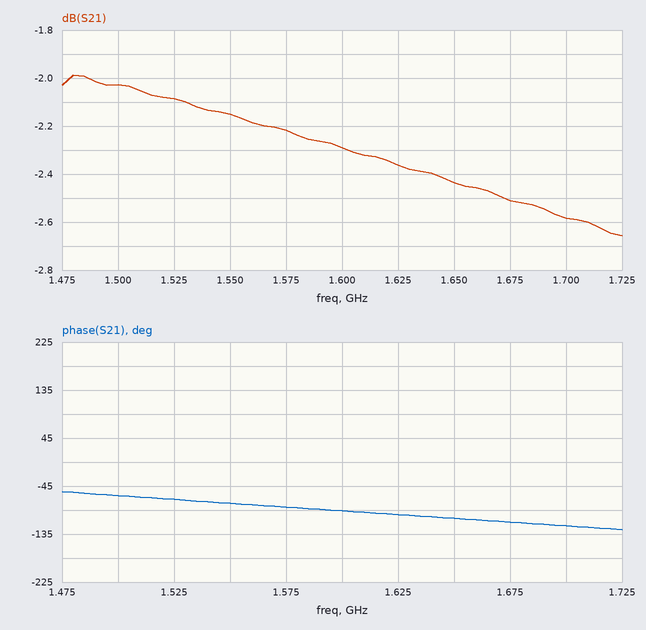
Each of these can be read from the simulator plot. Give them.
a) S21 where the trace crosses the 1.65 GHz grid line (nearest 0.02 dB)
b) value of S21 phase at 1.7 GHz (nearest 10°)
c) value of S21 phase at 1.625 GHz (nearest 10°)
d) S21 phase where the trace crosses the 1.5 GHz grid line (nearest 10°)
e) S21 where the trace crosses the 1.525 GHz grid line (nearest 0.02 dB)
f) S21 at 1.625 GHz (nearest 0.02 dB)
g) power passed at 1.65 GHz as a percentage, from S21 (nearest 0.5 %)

-2.44 dB
-120°
-100°
-60°
-2.08 dB
-2.36 dB
57.0 %
